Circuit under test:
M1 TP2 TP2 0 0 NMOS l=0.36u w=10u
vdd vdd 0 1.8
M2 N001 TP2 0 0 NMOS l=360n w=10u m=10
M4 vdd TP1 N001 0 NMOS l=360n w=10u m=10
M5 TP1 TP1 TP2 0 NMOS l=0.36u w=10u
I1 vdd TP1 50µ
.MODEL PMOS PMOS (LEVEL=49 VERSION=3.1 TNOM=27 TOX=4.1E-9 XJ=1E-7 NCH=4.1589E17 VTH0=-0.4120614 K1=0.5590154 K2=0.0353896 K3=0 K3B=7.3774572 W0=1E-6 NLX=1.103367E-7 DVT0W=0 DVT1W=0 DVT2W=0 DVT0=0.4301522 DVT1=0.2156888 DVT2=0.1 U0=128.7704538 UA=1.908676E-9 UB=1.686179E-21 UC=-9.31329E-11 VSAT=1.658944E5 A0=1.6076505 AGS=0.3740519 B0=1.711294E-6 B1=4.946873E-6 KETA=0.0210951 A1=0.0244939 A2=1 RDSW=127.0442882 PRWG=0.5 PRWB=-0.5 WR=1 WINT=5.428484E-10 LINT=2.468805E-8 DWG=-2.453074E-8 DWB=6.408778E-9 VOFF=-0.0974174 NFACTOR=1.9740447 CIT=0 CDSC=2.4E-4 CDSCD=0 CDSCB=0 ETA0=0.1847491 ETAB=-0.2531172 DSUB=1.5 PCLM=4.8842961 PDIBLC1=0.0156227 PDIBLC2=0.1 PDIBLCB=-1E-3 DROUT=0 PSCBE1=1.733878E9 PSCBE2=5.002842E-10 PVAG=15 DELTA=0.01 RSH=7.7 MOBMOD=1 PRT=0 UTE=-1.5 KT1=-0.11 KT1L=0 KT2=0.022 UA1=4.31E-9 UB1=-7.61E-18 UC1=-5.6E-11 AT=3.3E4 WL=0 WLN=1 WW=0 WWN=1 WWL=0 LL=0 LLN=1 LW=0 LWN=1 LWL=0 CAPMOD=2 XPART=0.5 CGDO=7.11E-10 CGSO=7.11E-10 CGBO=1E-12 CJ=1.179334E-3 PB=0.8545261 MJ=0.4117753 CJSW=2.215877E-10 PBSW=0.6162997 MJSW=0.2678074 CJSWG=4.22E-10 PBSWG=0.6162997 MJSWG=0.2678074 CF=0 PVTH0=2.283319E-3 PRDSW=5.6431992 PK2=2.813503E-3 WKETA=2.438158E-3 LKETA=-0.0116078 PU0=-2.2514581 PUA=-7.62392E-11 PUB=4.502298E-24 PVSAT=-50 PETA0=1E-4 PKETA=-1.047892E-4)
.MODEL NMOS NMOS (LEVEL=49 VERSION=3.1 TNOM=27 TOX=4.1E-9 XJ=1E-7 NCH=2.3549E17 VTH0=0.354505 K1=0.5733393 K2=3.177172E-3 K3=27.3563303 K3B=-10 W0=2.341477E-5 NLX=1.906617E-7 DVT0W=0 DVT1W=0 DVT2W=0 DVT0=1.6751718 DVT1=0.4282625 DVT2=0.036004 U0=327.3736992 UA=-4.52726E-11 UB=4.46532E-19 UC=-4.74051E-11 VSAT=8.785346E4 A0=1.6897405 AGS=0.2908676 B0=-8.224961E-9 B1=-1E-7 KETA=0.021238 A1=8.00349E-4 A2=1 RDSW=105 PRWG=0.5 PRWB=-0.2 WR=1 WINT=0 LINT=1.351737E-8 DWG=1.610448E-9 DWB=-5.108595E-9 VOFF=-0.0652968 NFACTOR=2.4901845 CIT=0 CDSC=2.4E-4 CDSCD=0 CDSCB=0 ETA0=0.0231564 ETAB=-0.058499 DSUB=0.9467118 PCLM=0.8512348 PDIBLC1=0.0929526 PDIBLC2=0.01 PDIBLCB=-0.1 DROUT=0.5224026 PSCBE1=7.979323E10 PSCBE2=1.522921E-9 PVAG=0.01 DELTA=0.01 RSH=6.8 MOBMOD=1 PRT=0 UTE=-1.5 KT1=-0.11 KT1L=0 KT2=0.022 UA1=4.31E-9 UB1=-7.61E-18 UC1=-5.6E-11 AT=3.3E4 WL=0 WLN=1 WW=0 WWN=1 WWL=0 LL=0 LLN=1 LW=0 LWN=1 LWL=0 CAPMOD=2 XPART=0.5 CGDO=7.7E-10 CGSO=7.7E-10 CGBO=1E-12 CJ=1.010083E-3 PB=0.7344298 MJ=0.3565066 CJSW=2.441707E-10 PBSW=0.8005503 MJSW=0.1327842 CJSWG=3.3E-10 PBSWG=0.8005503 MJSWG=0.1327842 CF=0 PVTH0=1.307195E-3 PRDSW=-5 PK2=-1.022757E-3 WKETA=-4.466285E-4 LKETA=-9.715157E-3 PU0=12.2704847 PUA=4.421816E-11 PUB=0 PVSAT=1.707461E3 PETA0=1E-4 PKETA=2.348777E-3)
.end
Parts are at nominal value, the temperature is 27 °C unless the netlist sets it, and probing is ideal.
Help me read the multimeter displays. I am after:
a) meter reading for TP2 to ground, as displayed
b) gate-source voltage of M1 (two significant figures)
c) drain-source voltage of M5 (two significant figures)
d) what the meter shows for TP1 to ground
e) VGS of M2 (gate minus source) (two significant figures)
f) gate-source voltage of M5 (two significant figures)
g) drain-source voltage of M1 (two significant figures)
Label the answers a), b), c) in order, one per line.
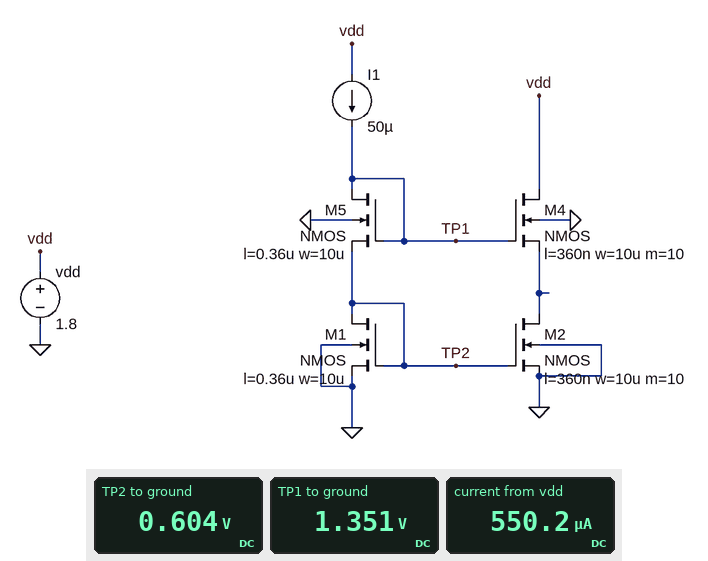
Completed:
a) 0.604 V
b) 600 mV
c) 750 mV
d) 1.351 V
e) 600 mV
f) 750 mV
g) 600 mV
